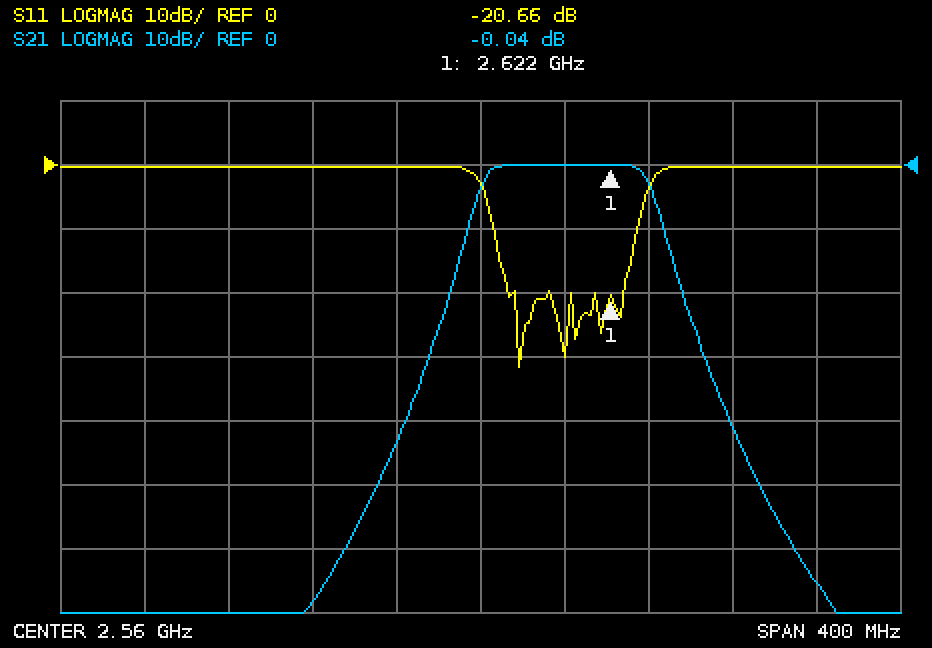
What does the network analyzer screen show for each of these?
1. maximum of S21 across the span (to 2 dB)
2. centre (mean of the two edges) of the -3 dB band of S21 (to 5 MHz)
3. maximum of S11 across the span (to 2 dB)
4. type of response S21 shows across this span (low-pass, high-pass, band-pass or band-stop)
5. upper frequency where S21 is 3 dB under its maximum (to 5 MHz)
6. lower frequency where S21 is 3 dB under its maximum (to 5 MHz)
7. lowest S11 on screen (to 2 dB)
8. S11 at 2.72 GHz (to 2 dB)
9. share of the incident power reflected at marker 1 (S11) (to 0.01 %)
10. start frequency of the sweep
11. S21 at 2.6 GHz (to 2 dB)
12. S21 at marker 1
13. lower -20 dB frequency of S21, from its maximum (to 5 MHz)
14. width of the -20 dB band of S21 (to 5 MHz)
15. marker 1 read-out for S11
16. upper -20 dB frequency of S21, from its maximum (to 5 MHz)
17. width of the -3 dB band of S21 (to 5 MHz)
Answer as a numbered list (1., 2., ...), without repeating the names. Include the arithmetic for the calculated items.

1. 0 dB
2. 2.600 GHz
3. 0 dB
4. band-pass
5. 2.640 GHz
6. 2.560 GHz
7. -32 dB
8. 0 dB
9. 10^(-20.66/10) ≈ 0.86 %
10. 2.36 GHz
11. 0 dB
12. -0.04 dB
13. 2.545 GHz
14. 2.655 GHz − 2.545 GHz = 110 MHz
15. -20.66 dB
16. 2.655 GHz
17. 2.640 GHz − 2.560 GHz = 80 MHz
